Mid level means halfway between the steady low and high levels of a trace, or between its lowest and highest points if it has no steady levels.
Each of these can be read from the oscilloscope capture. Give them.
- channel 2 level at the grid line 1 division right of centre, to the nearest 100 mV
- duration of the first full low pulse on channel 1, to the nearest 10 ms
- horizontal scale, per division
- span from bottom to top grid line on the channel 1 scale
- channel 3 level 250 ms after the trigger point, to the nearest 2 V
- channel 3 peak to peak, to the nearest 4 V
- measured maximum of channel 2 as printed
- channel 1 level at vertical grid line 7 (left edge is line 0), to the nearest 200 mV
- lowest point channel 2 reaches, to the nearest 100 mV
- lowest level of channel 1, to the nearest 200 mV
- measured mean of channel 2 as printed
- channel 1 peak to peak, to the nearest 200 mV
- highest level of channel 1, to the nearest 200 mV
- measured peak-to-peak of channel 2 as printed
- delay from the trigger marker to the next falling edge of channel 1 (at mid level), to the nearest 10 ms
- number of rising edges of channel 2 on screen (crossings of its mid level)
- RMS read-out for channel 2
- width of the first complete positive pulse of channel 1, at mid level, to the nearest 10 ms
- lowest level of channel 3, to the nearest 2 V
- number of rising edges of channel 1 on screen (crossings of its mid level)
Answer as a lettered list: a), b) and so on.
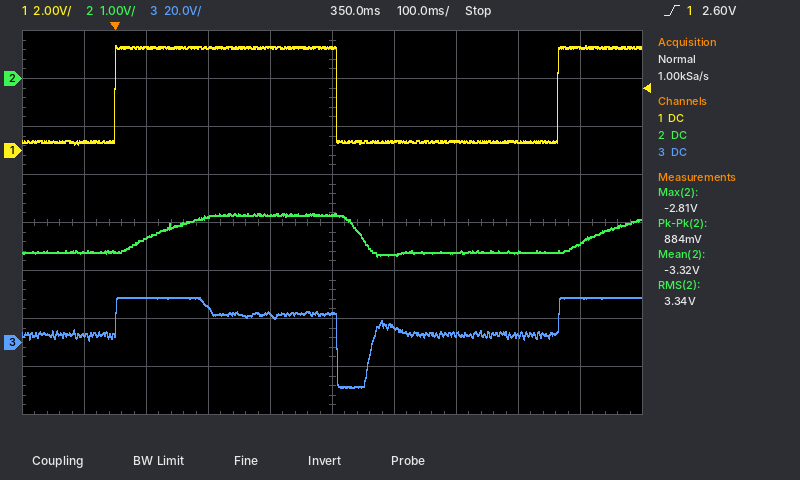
a) -3.7 V
b) 360 ms
c) 100 ms
d) 16 V
e) 12 V
f) 36 V
g) -2.81 V
h) 400 mV
i) -3.7 V
j) 200 mV
k) -3.32 V
l) 4.2 V
m) 4.4 V
n) 884 mV
o) 360 ms
p) 2
q) 3.34 V
r) 360 ms
s) -18 V
t) 2
